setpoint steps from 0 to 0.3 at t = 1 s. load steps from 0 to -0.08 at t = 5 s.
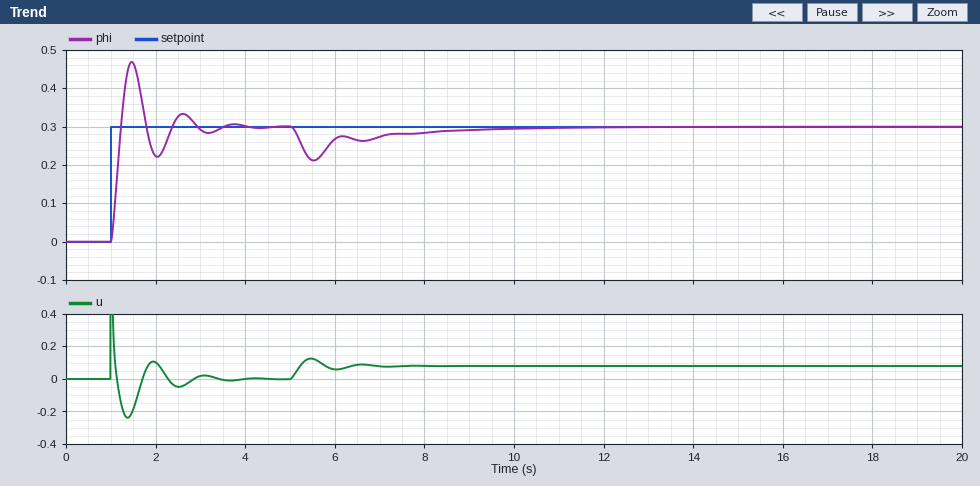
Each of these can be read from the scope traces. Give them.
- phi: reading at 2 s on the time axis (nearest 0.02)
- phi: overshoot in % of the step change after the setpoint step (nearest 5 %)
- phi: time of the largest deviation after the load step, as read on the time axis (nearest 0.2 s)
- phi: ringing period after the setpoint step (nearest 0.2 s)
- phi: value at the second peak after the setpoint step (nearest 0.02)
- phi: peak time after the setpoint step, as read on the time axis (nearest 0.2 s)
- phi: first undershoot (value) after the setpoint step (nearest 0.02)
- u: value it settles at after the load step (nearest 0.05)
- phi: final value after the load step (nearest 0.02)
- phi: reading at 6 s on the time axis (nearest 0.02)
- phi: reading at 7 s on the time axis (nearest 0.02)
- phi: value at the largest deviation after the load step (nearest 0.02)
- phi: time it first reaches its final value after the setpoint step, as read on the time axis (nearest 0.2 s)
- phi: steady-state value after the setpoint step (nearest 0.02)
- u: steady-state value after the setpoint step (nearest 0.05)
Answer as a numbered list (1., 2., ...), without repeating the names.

1. 0.22
2. 55 %
3. 5.6 s
4. 1.2 s
5. 0.34
6. 1.4 s
7. 0.22
8. 0.10
9. 0.30
10. 0.26
11. 0.28
12. 0.22
13. 1.2 s
14. 0.30
15. 0.00
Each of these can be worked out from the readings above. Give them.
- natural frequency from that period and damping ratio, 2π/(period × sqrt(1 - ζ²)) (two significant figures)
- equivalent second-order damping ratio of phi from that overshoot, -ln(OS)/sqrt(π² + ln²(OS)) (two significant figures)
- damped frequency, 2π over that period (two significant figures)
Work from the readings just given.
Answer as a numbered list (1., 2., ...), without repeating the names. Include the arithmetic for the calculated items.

1. 2π / (1.2 × sqrt(1 - 0.19²)) = 5.3 rad/s
2. ln(0.55) = -0.598; 0.598 / sqrt(9.870 + 0.357) = 0.19
3. 2π / 1.2 = 5.2 rad/s
